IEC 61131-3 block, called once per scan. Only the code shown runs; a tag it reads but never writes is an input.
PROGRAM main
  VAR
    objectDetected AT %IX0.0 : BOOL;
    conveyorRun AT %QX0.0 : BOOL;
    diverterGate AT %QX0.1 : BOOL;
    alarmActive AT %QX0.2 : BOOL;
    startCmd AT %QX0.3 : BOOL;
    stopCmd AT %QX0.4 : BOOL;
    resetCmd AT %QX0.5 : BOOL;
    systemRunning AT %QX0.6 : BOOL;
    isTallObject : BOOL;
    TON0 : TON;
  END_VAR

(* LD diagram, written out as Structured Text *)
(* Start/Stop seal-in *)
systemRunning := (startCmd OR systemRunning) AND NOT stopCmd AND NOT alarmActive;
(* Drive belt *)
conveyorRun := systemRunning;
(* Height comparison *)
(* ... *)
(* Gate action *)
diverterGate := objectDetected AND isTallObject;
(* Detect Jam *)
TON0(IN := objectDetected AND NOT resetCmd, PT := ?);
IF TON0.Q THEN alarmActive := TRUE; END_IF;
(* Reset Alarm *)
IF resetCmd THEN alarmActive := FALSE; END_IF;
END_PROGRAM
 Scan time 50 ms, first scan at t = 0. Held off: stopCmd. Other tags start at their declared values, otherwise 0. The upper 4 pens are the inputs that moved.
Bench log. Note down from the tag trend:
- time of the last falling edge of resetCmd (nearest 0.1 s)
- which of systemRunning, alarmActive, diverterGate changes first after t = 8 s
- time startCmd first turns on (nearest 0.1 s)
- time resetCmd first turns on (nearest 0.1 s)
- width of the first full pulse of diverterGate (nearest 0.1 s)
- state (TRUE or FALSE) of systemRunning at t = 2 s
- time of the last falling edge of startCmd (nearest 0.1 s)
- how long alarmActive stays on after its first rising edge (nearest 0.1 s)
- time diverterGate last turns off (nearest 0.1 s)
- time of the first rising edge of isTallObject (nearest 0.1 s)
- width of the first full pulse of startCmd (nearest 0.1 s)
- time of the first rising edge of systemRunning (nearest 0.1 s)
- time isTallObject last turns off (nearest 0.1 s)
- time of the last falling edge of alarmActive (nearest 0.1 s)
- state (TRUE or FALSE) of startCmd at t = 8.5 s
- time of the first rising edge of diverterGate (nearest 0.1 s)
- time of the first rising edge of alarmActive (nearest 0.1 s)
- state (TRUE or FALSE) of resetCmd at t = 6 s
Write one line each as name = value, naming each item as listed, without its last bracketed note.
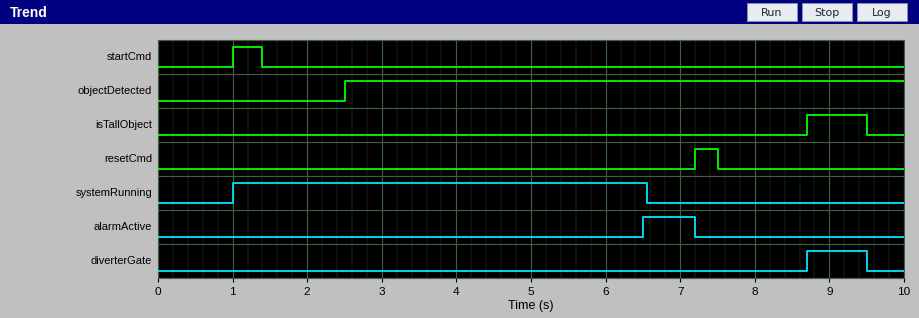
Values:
time of the last falling edge of resetCmd = 7.5 s
which of systemRunning, alarmActive, diverterGate changes first after t = 8 s = diverterGate
time startCmd first turns on = 1.0 s
time resetCmd first turns on = 7.2 s
width of the first full pulse of diverterGate = 0.8 s
state (TRUE or FALSE) of systemRunning at t = 2 s = TRUE
time of the last falling edge of startCmd = 1.4 s
how long alarmActive stays on after its first rising edge = 0.7 s
time diverterGate last turns off = 9.5 s
time of the first rising edge of isTallObject = 8.7 s
width of the first full pulse of startCmd = 0.4 s
time of the first rising edge of systemRunning = 1.0 s
time isTallObject last turns off = 9.5 s
time of the last falling edge of alarmActive = 7.2 s
state (TRUE or FALSE) of startCmd at t = 8.5 s = FALSE
time of the first rising edge of diverterGate = 8.7 s
time of the first rising edge of alarmActive = 6.5 s
state (TRUE or FALSE) of resetCmd at t = 6 s = FALSE
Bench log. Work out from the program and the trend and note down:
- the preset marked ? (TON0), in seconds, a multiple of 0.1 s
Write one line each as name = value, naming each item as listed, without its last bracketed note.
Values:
the preset marked ? (TON0), in seconds, a multiple of 0.1 s = 4.0 s
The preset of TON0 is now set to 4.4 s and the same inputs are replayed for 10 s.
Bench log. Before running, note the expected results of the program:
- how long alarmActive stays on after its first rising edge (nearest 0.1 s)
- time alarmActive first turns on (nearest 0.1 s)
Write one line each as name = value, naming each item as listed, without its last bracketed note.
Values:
how long alarmActive stays on after its first rising edge = 0.3 s
time alarmActive first turns on = 6.9 s
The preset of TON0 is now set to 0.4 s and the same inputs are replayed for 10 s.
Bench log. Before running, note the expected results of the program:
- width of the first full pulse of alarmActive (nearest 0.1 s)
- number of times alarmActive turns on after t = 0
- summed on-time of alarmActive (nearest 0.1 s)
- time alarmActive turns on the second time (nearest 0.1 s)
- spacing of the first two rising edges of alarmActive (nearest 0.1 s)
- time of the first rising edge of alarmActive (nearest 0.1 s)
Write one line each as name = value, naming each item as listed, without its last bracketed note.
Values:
width of the first full pulse of alarmActive = 4.3 s
number of times alarmActive turns on after t = 0 = 2
summed on-time of alarmActive = 6.4 s
time alarmActive turns on the second time = 7.9 s
spacing of the first two rising edges of alarmActive = 5.0 s
time of the first rising edge of alarmActive = 2.9 s
